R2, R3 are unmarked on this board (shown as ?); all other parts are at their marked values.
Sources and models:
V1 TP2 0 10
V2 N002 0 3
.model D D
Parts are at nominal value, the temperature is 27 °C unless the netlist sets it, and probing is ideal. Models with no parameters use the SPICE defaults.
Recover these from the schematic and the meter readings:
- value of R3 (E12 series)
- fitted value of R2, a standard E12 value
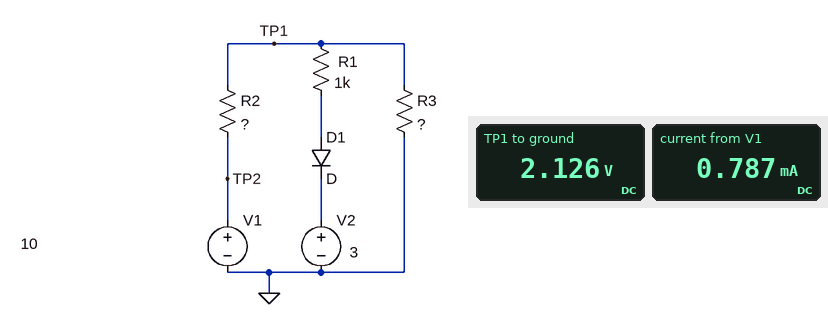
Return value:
2.7 kΩ
10 kΩ
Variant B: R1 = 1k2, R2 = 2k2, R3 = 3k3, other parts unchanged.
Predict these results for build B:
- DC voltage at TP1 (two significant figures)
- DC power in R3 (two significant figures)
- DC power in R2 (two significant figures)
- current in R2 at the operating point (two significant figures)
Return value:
4.8 V
6.9 mW
12 mW
2.4 mA
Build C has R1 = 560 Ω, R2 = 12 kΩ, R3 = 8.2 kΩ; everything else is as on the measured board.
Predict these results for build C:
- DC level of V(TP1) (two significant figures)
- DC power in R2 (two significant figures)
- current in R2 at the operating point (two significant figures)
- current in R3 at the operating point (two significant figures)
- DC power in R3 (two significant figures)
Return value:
3.6 V
3.4 mW
530 µA
440 µA
1.6 mW
